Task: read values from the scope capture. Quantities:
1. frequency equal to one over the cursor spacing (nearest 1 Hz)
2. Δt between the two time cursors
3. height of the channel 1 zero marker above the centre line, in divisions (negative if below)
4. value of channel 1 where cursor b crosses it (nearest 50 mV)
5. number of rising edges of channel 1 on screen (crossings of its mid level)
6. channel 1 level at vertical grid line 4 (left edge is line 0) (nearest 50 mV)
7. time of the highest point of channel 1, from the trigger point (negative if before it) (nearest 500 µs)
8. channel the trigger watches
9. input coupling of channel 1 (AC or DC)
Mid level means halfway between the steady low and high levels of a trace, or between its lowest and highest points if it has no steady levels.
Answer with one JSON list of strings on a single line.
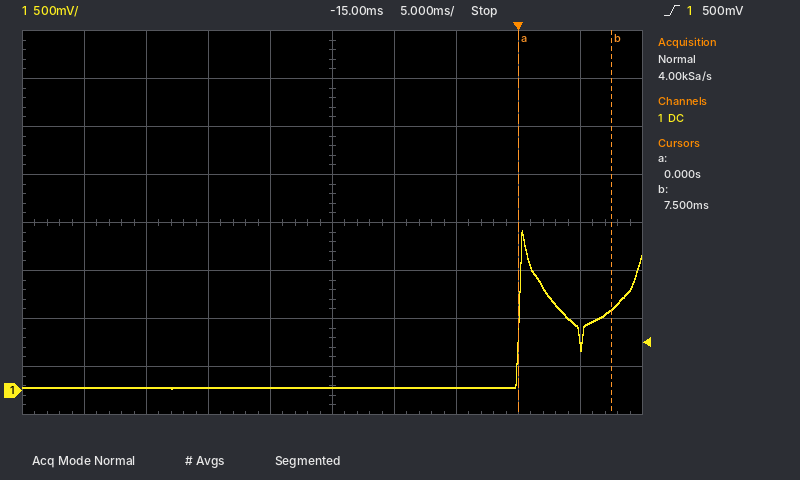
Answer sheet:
["133 Hz", "7.5 ms", "-3.5 div", "850 mV", "2", "50 mV", "+500 µs", "channel 1", "DC"]
